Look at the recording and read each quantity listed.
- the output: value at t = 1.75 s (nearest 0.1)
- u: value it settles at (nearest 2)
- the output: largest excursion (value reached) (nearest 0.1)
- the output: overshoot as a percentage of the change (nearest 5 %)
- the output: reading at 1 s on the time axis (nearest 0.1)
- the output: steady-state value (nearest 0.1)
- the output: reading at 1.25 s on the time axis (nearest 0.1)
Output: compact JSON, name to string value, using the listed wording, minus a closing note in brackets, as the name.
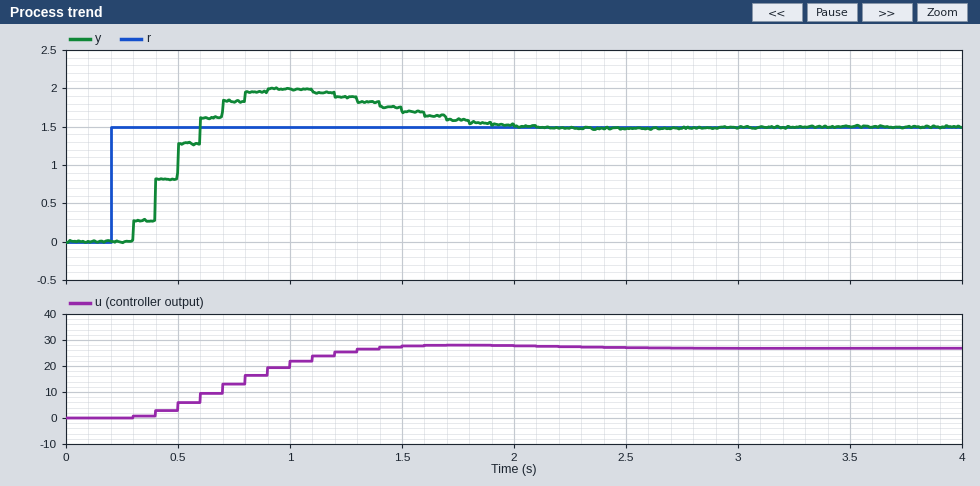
{"the output: value at t = 1.75 s": "1.6", "u: value it settles at": "26", "the output: largest excursion (value reached)": "2.0", "the output: overshoot as a percentage of the change": "35 %", "the output: reading at 1 s on the time axis": "2.0", "the output: steady-state value": "1.5", "the output: reading at 1.25 s on the time axis": "1.9"}
